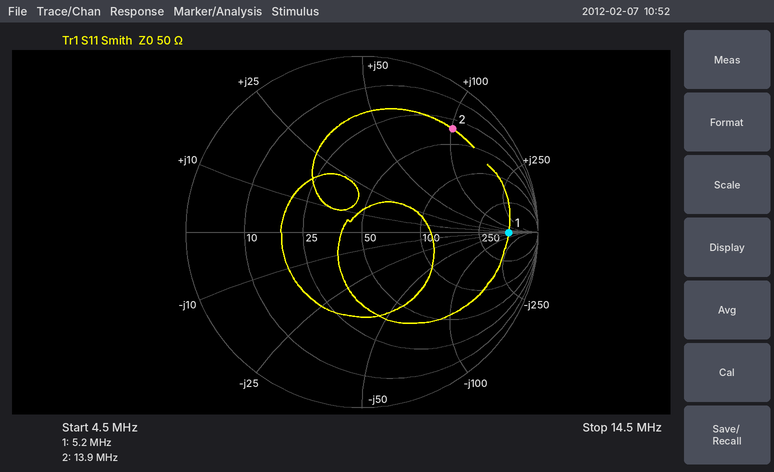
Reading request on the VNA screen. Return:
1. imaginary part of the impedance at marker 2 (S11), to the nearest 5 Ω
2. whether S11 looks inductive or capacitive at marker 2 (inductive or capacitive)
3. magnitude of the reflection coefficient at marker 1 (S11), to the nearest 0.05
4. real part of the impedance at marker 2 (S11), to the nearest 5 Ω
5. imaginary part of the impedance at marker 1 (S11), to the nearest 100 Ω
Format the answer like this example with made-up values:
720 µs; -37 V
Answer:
+100 Ω; inductive; 0.85; 35 Ω; 0 Ω
